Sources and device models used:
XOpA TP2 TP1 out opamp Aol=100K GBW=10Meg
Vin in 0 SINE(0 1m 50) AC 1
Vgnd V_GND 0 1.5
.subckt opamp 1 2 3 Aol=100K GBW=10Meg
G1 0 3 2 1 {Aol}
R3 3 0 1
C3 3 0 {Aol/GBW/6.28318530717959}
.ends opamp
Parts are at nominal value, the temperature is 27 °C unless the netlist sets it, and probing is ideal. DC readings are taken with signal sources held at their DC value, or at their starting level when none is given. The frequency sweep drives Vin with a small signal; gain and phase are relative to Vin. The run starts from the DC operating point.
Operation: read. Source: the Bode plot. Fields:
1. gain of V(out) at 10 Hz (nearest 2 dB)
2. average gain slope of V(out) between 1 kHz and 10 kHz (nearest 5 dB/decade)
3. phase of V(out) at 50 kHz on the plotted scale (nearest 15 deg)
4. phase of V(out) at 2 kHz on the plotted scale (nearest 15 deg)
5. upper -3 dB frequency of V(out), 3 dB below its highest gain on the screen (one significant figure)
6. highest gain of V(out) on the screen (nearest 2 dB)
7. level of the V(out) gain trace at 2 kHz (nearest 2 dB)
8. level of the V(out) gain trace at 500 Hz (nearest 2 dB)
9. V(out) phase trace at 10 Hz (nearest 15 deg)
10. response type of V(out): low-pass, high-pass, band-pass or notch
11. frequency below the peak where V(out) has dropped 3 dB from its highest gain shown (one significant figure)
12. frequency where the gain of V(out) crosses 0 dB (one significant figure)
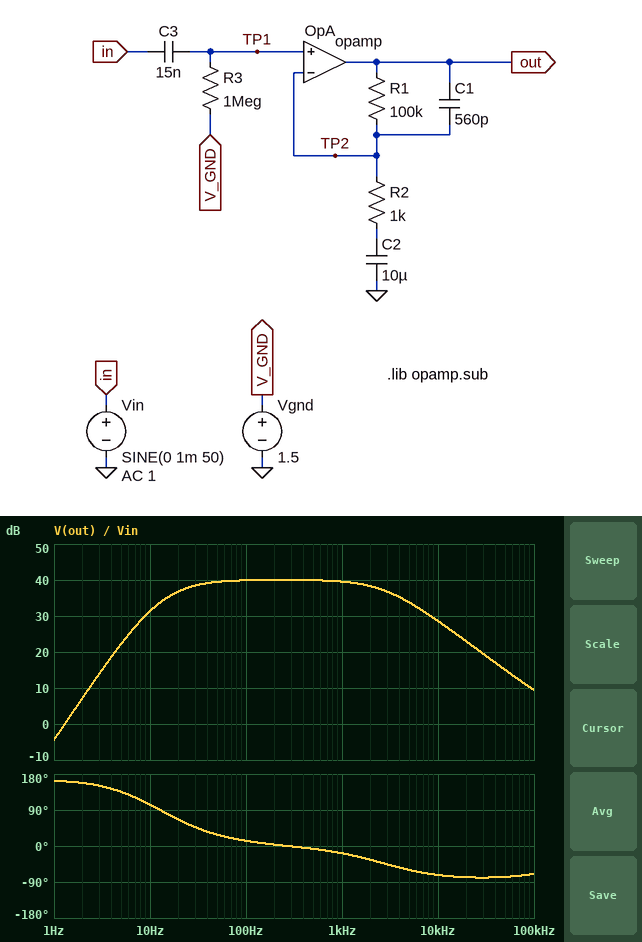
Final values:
32 dB
-10 dB/decade
-75 deg
-30 deg
3 kHz
40 dB
38 dB
40 dB
105 deg
band-pass
20 Hz
1 Hz
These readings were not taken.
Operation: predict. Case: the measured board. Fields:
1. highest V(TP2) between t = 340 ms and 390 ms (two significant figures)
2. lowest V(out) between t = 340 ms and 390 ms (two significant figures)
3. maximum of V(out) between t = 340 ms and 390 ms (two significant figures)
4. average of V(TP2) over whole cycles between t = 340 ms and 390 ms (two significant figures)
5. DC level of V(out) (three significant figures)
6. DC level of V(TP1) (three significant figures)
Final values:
1.5 V
1.4 V
1.6 V
1.5 V
1.50 V
1.50 V
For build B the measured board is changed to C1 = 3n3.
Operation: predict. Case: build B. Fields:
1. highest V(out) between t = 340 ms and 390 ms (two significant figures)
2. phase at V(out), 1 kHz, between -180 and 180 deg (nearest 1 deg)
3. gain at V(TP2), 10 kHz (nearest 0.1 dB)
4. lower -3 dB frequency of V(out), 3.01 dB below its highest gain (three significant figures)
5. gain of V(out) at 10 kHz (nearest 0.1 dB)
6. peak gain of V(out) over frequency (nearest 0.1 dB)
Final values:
1.6 V
-62 deg
0 dB
19.5 Hz
13.9 dB
39.7 dB
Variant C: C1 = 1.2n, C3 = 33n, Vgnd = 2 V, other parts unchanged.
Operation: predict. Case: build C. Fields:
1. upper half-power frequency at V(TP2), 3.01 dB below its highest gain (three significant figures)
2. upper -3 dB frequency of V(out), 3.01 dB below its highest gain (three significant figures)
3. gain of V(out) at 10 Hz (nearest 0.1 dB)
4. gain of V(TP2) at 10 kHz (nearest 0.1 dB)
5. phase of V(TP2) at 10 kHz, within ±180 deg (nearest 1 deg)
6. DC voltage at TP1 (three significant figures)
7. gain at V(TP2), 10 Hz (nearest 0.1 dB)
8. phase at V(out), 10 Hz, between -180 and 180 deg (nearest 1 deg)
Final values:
9.89 MHz
1.34 kHz
33.7 dB
-0.1 dB
0 deg
2.00 V
-0.9 dB
82 deg
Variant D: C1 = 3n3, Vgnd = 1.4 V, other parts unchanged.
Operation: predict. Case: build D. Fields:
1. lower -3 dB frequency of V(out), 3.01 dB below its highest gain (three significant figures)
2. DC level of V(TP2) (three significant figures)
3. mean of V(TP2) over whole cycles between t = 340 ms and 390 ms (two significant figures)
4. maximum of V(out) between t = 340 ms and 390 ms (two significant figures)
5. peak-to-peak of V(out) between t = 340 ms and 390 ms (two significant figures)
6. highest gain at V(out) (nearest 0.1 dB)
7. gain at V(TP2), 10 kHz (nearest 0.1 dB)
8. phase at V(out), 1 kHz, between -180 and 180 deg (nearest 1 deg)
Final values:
19.5 Hz
1.40 V
1.4 V
1.5 V
190 mV
39.7 dB
0 dB
-62 deg
